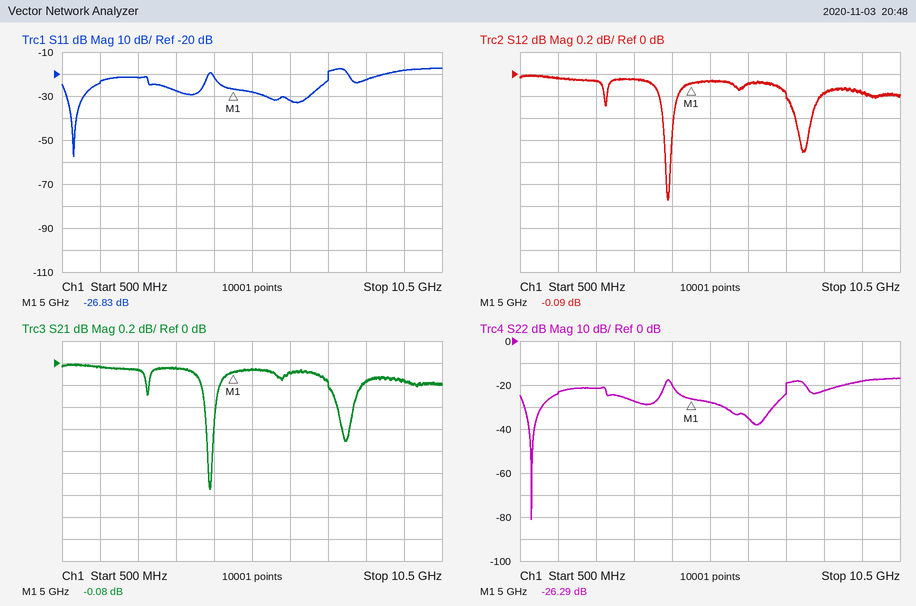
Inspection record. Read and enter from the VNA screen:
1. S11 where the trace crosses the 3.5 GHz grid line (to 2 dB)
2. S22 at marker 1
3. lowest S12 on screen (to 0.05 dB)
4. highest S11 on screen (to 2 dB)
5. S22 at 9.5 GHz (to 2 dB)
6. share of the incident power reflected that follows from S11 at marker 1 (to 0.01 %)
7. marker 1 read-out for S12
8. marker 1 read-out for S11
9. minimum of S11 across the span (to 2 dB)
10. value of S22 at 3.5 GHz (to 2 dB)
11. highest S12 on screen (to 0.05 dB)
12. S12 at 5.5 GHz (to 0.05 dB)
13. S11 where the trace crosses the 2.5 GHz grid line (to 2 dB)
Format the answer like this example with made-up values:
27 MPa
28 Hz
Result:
-28 dB
-26.29 dB
-1.15 dB
-18 dB
-18 dB
0.21 %
-0.09 dB
-26.83 dB
-58 dB
-28 dB
0.00 dB
-0.05 dB
-22 dB
